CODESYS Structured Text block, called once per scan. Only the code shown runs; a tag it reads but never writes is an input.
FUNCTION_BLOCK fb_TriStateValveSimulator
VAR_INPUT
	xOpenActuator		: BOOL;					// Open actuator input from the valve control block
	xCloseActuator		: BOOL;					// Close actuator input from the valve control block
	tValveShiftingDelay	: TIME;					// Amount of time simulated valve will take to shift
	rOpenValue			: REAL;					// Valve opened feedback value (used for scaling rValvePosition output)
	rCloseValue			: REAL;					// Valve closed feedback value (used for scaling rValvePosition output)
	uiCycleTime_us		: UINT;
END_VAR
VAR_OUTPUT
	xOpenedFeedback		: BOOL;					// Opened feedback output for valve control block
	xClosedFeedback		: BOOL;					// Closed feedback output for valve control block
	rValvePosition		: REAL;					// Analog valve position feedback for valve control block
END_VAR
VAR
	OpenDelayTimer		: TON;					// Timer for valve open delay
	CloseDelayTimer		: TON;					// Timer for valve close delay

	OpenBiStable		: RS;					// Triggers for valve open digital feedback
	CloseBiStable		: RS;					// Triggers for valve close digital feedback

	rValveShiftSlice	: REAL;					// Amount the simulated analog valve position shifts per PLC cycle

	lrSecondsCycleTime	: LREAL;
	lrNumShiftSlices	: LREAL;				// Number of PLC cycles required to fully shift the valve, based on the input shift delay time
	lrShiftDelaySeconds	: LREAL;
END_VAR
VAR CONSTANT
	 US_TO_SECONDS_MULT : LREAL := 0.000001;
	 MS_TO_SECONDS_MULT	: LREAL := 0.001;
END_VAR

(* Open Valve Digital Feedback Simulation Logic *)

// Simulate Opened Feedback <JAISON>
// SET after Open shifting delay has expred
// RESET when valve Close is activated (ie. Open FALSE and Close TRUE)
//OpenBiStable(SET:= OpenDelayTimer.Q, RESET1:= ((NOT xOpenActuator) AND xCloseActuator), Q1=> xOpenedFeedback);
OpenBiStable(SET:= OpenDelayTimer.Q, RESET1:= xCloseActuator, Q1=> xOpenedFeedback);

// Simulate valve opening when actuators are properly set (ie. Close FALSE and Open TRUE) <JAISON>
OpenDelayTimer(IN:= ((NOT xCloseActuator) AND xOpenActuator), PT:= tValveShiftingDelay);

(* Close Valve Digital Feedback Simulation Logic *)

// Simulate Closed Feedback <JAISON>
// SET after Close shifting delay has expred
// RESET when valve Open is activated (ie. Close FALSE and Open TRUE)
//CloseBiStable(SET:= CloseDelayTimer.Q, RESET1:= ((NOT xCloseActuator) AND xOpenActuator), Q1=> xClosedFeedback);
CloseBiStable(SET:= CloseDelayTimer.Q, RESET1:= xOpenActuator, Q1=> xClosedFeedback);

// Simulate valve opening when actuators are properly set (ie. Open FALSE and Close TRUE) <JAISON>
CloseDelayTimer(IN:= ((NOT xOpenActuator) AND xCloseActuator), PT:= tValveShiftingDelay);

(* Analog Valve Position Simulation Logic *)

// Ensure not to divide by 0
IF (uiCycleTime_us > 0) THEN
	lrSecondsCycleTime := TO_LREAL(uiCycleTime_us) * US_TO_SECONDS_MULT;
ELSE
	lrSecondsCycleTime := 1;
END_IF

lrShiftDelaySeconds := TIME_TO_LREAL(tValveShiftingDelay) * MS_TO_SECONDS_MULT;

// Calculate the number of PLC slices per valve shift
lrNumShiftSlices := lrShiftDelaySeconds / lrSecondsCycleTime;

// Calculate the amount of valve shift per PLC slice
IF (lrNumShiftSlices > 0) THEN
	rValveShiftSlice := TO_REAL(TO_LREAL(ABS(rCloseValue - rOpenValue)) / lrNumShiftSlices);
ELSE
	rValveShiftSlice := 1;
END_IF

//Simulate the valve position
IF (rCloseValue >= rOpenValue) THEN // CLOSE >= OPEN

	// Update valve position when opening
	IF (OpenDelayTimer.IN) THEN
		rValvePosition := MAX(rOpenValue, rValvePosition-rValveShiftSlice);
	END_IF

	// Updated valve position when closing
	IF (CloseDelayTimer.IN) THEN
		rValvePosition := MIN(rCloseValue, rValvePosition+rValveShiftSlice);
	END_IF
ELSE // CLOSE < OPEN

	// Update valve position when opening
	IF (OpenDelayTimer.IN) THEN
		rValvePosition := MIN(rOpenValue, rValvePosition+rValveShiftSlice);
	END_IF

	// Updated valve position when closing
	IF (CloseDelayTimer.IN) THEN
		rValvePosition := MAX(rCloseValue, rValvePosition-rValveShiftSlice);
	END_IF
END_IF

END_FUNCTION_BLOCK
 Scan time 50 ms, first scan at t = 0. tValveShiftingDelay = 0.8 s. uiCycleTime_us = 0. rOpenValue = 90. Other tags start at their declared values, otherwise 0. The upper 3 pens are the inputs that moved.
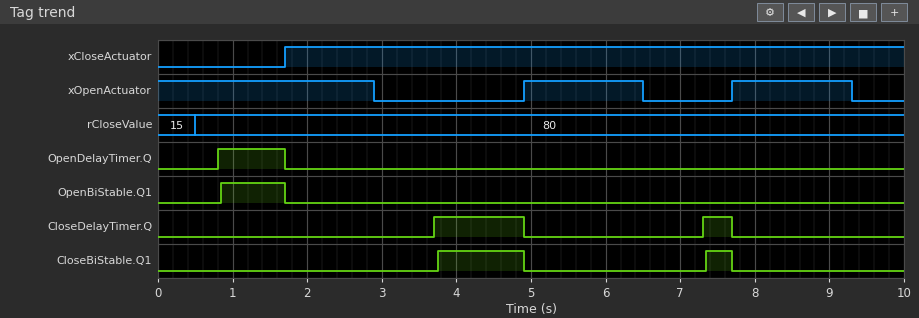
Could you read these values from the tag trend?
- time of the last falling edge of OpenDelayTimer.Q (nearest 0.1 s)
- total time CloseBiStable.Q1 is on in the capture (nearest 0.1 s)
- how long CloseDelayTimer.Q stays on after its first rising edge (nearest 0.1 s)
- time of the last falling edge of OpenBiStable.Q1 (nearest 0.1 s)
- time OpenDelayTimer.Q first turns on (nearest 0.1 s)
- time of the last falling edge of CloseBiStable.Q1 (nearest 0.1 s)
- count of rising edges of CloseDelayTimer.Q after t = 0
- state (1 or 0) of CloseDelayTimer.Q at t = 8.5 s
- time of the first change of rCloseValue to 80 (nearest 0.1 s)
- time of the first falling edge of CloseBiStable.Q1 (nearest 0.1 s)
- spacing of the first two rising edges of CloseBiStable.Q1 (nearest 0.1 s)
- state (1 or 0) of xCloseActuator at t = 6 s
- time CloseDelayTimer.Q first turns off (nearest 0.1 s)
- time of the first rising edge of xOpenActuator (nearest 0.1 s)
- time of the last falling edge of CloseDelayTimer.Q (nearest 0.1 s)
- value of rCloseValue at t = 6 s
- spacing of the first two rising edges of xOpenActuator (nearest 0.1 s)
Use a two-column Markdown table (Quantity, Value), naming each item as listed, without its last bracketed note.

| Quantity | Value |
|---|---|
| time of the last falling edge of OpenDelayTimer.Q | 1.7 s |
| total time CloseBiStable.Q1 is on in the capture | 1.5 s |
| how long CloseDelayTimer.Q stays on after its first rising edge | 1.2 s |
| time of the last falling edge of OpenBiStable.Q1 | 1.7 s |
| time OpenDelayTimer.Q first turns on | 0.8 s |
| time of the last falling edge of CloseBiStable.Q1 | 7.7 s |
| count of rising edges of CloseDelayTimer.Q after t = 0 | 2 |
| state (1 or 0) of CloseDelayTimer.Q at t = 8.5 s | 0 |
| time of the first change of rCloseValue to 80 | 0.5 s |
| time of the first falling edge of CloseBiStable.Q1 | 4.9 s |
| spacing of the first two rising edges of CloseBiStable.Q1 | 3.6 s |
| state (1 or 0) of xCloseActuator at t = 6 s | 1 |
| time CloseDelayTimer.Q first turns off | 4.9 s |
| time of the first rising edge of xOpenActuator | 4.9 s |
| time of the last falling edge of CloseDelayTimer.Q | 7.7 s |
| value of rCloseValue at t = 6 s | 80 |
| spacing of the first two rising edges of xOpenActuator | 2.8 s |
